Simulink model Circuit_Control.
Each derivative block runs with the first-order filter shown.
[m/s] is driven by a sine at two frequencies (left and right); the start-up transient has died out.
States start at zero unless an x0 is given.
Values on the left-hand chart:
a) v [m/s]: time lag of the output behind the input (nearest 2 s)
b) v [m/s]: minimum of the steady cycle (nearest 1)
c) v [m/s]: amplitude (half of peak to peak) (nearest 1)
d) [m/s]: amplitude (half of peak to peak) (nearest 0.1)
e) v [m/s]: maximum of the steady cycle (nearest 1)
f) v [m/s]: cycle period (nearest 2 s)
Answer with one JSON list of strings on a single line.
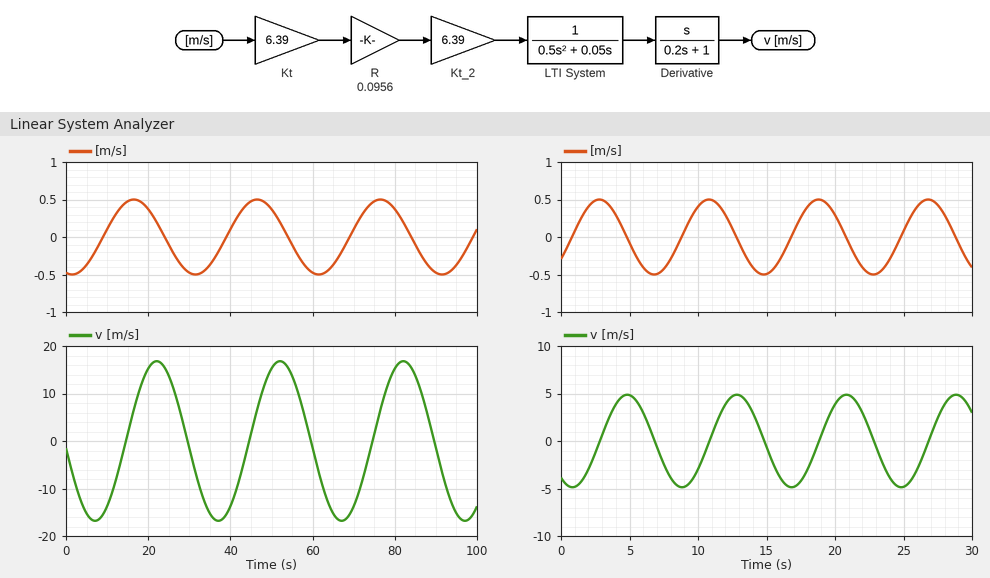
["6 s", "-17", "17", "0.5", "17", "30 s"]
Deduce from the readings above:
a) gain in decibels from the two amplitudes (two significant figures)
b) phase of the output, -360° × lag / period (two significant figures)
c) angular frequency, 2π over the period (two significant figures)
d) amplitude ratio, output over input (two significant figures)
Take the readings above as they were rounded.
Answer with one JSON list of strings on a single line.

["31 dB", "-72°", "0.21 rad/s", "34"]
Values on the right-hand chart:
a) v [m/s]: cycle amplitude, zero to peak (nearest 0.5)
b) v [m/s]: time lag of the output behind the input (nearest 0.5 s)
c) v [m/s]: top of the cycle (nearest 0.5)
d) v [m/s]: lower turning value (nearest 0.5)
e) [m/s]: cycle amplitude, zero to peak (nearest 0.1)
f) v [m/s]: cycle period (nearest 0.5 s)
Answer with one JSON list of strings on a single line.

["5.0", "2.0 s", "5.0", "-5.0", "0.5", "8.0 s"]
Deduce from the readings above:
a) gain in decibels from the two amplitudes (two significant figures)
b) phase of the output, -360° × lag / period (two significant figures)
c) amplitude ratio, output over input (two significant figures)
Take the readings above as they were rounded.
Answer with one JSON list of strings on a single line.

["20 dB", "-90°", "10"]
